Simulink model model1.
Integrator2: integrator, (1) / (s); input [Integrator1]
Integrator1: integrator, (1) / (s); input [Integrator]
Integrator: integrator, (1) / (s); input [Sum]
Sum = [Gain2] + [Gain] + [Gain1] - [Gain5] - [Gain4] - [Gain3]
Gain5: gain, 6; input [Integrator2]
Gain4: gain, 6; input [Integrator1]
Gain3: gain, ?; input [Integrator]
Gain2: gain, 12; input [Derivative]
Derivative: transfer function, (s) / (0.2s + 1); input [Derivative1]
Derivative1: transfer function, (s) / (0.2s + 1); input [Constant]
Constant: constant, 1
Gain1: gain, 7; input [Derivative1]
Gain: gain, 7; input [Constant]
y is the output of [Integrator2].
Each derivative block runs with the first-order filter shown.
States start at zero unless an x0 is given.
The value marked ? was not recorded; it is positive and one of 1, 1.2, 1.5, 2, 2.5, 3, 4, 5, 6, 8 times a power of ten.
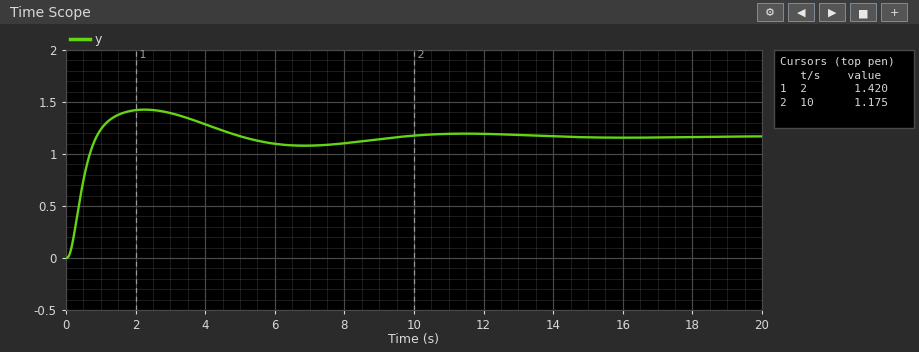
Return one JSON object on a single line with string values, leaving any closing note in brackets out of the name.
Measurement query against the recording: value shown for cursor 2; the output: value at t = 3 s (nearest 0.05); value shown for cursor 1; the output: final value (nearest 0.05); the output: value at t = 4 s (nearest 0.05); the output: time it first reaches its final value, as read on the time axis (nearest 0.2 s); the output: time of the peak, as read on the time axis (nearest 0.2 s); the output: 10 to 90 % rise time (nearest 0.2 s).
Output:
{"value shown for cursor 2": "1.175", "the output: value at t = 3 s": "1.40", "value shown for cursor 1": "1.420", "the output: final value": "1.15", "the output: value at t = 4 s": "1.30", "the output: time it first reaches its final value, as read on the time axis": "0.8 s", "the output: time of the peak, as read on the time axis": "2.2 s", "the output: 10 to 90 % rise time": "0.6 s"}
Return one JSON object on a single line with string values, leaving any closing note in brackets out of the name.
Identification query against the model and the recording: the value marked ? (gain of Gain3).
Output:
{"the value marked ?": "12"}
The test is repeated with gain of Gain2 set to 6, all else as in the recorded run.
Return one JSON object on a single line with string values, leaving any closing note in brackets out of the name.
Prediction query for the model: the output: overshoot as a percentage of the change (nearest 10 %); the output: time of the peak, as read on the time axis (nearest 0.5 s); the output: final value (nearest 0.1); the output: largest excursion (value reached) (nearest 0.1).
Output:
{"the output: overshoot as a percentage of the change": "30 %", "the output: time of the peak, as read on the time axis": "3.5 s", "the output: final value": "1.2", "the output: largest excursion (value reached)": "1.5"}
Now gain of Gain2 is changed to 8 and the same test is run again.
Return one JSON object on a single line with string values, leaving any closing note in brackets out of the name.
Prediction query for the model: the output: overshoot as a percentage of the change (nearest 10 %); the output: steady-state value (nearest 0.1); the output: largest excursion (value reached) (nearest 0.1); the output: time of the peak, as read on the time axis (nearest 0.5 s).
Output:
{"the output: overshoot as a percentage of the change": "30 %", "the output: steady-state value": "1.2", "the output: largest excursion (value reached)": "1.5", "the output: time of the peak, as read on the time axis": "3.0 s"}
